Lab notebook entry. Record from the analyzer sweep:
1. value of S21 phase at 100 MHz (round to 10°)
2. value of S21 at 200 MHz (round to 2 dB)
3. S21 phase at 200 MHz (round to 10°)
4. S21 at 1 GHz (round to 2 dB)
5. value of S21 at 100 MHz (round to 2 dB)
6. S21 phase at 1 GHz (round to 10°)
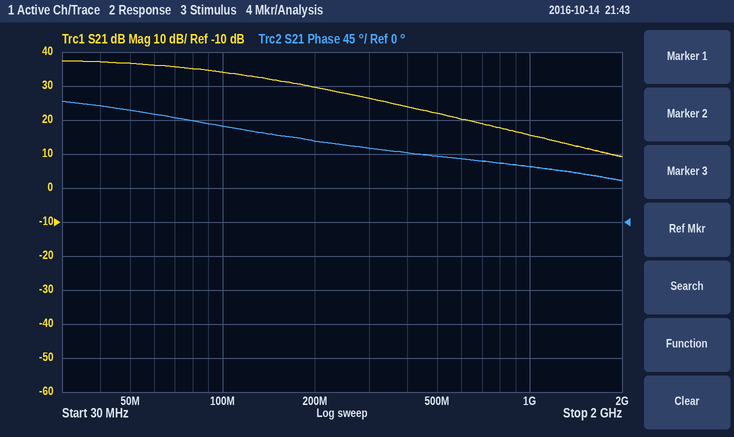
130°
30 dB
110°
16 dB
34 dB
70°
